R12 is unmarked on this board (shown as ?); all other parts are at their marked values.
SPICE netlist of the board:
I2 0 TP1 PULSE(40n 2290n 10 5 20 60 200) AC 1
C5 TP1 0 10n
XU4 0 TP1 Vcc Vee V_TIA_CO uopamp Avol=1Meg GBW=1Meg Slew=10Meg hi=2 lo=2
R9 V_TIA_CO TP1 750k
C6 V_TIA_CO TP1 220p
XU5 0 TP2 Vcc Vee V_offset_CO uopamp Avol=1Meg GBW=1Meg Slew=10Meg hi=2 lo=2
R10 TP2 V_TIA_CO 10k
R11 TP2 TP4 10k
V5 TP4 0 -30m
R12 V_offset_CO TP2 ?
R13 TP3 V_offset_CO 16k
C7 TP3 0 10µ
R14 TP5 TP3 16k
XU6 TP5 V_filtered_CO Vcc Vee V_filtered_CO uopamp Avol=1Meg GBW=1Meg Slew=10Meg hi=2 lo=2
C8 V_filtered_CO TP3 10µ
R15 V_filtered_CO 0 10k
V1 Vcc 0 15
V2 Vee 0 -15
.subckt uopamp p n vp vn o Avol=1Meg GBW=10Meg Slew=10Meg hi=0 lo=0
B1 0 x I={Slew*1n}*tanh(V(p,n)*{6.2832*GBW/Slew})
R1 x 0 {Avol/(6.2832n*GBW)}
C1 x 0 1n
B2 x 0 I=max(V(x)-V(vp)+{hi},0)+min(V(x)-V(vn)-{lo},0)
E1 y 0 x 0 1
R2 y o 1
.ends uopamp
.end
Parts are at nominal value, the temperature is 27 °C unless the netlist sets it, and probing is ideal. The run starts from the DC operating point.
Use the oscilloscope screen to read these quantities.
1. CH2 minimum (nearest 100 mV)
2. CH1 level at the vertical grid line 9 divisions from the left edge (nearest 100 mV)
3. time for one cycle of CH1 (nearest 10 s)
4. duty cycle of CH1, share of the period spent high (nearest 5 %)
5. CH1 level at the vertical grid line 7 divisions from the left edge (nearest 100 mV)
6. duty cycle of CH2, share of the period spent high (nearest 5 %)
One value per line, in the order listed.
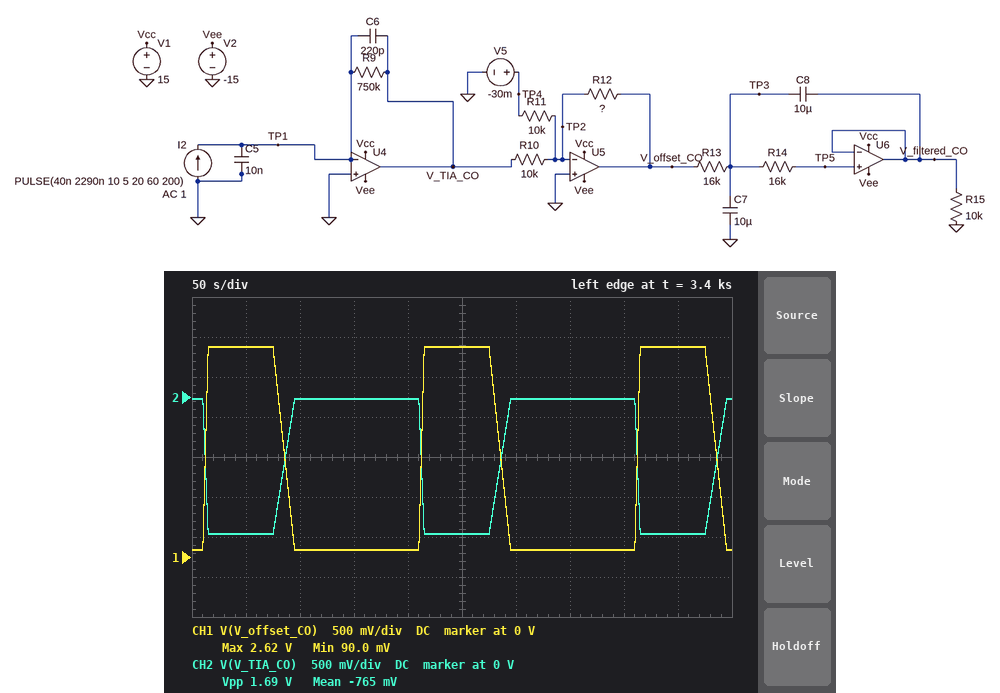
-1.7 V
2.6 V
200 s
35 %
100 mV
65 %
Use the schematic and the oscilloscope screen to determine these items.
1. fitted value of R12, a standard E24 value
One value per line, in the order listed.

15 kΩ
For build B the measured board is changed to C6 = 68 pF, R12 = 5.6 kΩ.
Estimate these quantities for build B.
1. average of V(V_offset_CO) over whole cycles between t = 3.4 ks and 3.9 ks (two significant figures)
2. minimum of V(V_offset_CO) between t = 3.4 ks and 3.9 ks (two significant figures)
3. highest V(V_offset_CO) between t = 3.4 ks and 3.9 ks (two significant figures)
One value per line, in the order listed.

380 mV
34 mV
980 mV
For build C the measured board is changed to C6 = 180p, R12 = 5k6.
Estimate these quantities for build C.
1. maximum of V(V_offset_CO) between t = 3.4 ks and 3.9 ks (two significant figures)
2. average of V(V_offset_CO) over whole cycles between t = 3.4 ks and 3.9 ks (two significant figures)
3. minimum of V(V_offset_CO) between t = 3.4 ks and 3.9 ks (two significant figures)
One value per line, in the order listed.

980 mV
380 mV
34 mV
